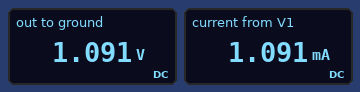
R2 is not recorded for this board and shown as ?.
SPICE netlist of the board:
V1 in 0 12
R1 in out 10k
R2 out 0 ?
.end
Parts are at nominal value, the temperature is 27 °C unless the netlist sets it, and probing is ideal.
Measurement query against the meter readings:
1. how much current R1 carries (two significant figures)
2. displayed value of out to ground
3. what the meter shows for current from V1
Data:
1.1 mA
1.091 V
1.091 mA
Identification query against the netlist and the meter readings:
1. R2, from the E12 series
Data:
1 kΩ
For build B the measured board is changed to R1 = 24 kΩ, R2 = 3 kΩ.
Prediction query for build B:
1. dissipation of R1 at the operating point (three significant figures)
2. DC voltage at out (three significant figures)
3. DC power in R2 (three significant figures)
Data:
4.74 mW
1.33 V
593 µW
